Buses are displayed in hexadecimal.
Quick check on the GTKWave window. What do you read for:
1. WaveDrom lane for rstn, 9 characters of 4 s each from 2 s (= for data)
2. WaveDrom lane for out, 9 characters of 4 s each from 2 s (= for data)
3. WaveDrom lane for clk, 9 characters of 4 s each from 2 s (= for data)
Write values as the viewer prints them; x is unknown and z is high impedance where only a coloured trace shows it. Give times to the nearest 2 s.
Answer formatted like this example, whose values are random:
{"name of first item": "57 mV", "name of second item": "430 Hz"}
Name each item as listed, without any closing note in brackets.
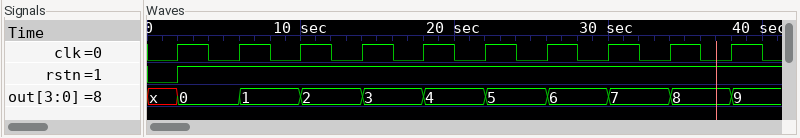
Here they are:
{"WaveDrom lane for rstn, 9 characters of 4 s each from 2 s": "{name: 'rstn', wave: '1........'}", "WaveDrom lane for out, 9 characters of 4 s each from 2 s": "{name: 'out', wave: '=========', data: '0 1 2 3 4 5 6 7 8'}", "WaveDrom lane for clk, 9 characters of 4 s each from 2 s": "{name: 'clk', wave: 'p........'}"}
